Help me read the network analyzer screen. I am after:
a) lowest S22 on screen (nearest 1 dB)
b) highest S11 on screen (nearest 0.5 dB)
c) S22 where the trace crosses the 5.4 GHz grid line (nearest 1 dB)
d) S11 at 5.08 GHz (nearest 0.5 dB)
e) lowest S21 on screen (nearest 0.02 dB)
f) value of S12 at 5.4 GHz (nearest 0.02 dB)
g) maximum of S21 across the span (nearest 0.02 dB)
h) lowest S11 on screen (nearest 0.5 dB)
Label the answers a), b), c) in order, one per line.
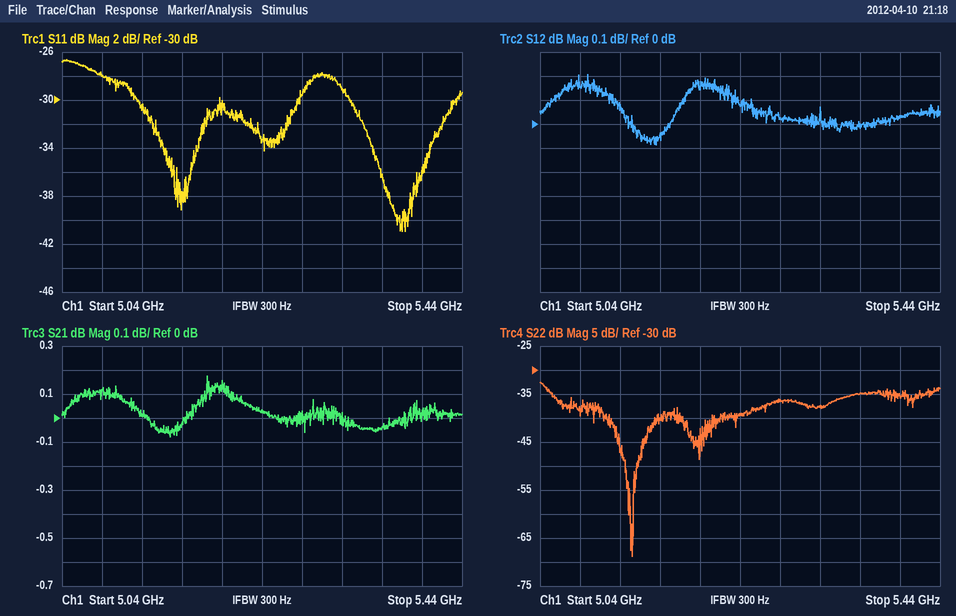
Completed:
a) -69 dB
b) -26.5 dB
c) -35 dB
d) -28.0 dB
e) -0.08 dB
f) 0.04 dB
g) 0.18 dB
h) -41.0 dB
